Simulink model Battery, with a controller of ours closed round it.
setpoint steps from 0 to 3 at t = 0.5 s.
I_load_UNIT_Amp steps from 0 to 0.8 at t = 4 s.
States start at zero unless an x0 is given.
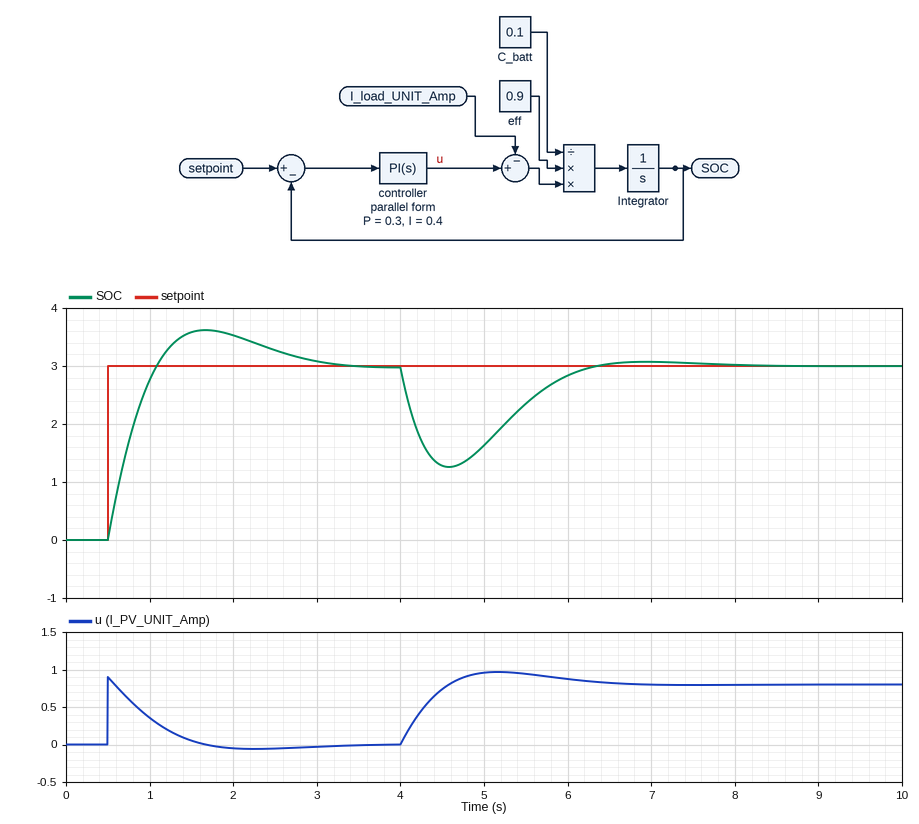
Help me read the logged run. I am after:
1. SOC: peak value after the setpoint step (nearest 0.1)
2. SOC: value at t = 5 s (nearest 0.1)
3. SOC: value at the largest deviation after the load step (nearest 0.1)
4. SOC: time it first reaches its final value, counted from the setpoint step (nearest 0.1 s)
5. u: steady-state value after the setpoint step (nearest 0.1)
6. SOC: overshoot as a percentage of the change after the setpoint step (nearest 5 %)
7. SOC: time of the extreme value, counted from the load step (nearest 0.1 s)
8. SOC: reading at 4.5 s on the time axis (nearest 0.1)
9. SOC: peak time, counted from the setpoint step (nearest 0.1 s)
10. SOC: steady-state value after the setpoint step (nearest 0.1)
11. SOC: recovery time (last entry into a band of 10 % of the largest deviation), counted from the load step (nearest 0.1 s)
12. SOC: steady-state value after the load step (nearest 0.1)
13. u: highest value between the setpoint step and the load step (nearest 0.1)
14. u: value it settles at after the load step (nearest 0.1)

3.6
1.6
1.3
0.6 s
0.0
20 %
0.6 s
1.3
1.2 s
3.0
2.0 s
3.0
0.9
0.8
